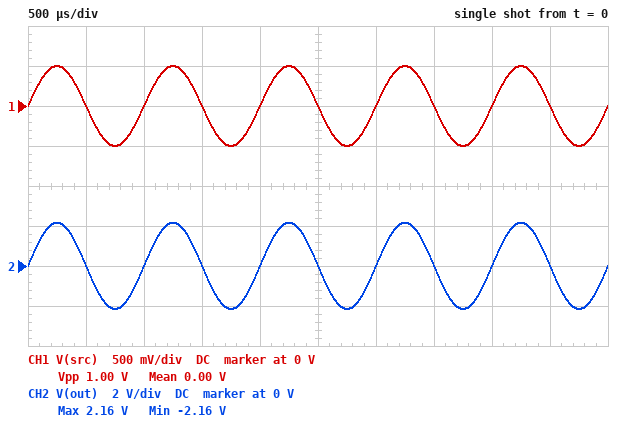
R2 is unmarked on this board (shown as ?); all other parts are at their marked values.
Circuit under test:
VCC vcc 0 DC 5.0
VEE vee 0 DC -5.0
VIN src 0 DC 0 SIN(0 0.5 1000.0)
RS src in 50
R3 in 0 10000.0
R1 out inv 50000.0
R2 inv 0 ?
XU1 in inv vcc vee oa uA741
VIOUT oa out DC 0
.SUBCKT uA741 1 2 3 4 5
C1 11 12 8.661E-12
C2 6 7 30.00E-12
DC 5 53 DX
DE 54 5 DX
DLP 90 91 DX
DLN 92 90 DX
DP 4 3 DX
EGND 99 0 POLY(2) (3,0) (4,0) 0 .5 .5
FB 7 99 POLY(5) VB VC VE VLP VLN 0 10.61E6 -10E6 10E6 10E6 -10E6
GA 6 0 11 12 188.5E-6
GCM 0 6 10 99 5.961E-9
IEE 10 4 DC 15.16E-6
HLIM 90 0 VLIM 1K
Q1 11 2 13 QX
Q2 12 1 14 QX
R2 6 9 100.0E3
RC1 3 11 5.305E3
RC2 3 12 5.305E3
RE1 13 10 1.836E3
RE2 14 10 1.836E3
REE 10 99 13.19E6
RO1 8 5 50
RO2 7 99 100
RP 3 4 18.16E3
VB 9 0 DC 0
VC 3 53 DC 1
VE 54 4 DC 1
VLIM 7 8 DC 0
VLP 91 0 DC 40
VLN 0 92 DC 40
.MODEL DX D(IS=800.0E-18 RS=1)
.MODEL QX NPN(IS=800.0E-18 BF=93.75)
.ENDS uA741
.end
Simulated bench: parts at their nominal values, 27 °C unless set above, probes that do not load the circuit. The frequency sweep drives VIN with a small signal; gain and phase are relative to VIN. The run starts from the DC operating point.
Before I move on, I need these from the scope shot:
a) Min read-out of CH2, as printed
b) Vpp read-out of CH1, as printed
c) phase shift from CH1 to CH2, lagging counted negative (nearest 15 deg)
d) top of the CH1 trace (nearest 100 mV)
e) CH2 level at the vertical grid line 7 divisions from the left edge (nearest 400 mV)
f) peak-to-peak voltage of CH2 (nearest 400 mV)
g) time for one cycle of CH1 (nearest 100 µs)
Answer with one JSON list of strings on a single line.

["-2.16 V", "1.00 V", "0 deg", "500 mV", "0 V", "4.4 V", "1.0 ms"]
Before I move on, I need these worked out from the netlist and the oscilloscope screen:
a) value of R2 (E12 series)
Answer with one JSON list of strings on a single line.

["15 kΩ"]
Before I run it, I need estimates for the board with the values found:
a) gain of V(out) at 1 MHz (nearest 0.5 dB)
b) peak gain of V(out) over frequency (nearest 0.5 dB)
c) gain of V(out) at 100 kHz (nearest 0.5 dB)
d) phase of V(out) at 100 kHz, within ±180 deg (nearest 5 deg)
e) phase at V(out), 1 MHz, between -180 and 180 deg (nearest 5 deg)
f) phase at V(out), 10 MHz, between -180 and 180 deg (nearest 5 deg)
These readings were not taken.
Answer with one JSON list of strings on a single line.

["-0.5 dB", "12.5 dB", "12.0 dB", "-25 deg", "-110 deg", "-170 deg"]
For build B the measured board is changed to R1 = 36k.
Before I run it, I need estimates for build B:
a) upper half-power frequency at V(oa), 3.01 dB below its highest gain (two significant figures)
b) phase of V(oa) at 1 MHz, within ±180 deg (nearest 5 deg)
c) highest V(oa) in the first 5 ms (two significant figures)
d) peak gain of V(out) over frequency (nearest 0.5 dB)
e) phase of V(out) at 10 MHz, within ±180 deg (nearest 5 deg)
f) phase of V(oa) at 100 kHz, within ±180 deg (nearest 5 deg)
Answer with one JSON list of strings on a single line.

["350 kHz", "-105 deg", "1.7 V", "10.5 dB", "-170 deg", "-20 deg"]
